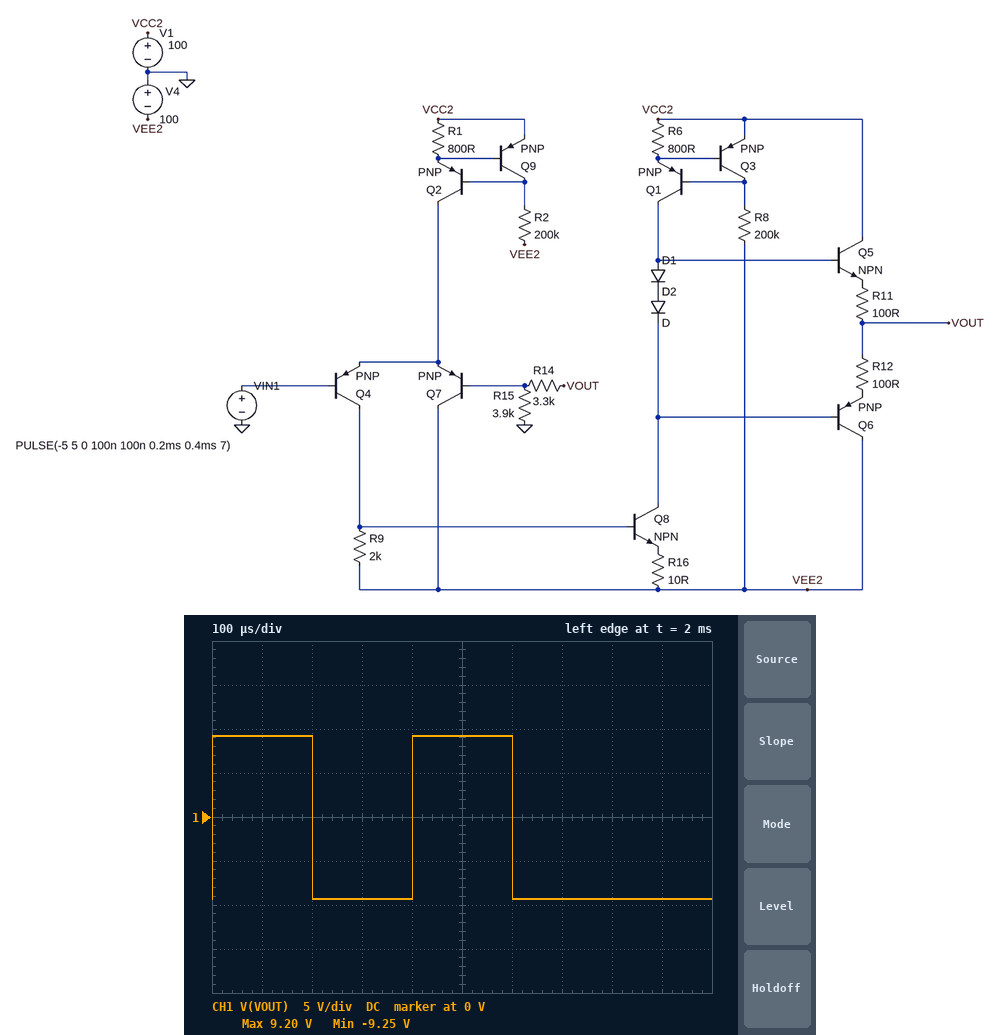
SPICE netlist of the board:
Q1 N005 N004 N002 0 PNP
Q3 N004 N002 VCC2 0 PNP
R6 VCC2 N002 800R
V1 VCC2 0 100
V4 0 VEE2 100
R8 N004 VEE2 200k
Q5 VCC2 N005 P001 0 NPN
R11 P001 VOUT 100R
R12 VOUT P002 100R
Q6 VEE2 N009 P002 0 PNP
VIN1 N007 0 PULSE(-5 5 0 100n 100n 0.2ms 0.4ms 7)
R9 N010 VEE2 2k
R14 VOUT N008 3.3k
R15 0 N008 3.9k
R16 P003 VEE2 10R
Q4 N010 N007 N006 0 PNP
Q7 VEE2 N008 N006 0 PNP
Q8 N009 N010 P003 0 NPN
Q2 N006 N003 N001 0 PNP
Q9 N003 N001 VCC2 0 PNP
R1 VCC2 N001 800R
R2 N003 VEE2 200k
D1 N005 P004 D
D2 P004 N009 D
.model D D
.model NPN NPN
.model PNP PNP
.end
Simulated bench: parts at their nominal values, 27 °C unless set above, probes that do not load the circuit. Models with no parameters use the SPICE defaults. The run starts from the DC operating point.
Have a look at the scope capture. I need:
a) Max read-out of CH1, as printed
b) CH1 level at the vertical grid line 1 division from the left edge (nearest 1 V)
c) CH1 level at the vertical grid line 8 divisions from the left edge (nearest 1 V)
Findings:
9.20 V
9 V
-9 V
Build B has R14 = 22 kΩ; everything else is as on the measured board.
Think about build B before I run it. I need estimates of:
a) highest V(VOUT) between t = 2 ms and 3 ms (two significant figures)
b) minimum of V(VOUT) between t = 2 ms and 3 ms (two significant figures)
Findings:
33 V
-33 V
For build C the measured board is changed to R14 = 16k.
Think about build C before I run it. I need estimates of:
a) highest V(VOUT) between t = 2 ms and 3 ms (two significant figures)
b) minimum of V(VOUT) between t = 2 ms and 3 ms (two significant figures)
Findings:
25 V
-26 V
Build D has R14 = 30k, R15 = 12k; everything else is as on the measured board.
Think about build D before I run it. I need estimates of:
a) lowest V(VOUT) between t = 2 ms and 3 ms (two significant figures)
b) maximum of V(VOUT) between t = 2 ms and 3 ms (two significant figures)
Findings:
-18 V
17 V
